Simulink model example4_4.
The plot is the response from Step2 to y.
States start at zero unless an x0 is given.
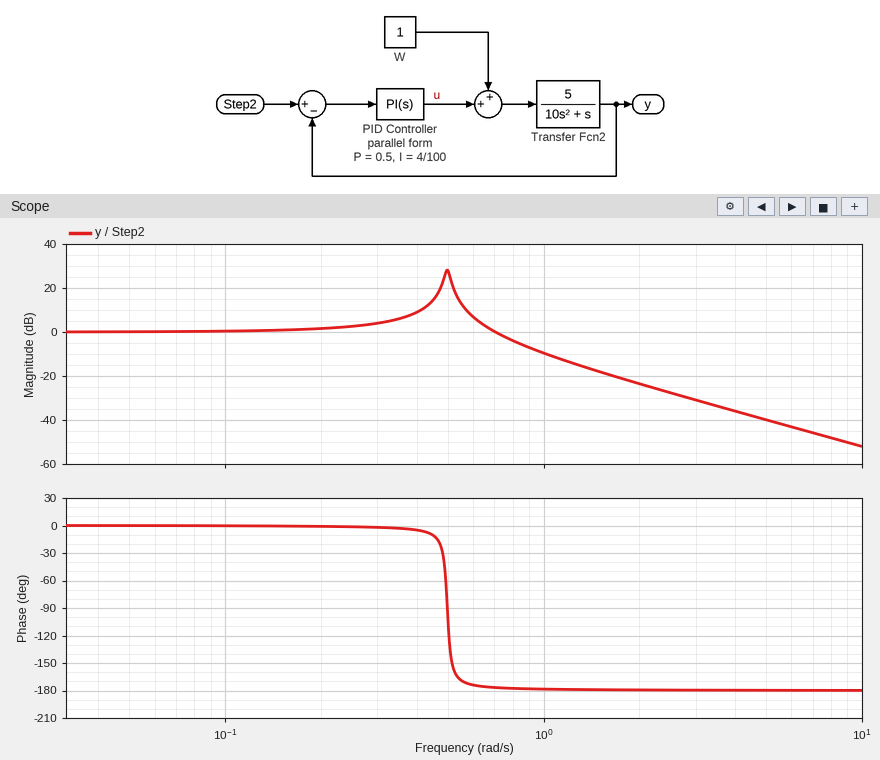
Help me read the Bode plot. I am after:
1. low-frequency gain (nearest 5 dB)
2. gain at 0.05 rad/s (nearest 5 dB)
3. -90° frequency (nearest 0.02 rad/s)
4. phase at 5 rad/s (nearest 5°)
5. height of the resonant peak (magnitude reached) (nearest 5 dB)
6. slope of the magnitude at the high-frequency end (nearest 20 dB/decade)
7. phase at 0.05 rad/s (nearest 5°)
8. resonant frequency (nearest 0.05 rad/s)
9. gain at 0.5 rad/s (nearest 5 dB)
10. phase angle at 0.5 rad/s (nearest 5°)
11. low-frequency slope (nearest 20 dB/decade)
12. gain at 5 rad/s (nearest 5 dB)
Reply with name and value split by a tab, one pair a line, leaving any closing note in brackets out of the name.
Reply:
low-frequency gain	0 dB
gain at 0.05 rad/s	0 dB
-90° frequency	0.50 rad/s
phase at 5 rad/s	-180°
height of the resonant peak (magnitude reached)	30 dB
slope of the magnitude at the high-frequency end	-40 dB/decade
phase at 0.05 rad/s	0°
resonant frequency	0.50 rad/s
gain at 0.5 rad/s	30 dB
phase angle at 0.5 rad/s	-100°
low-frequency slope	0 dB/decade
gain at 5 rad/s	-40 dB
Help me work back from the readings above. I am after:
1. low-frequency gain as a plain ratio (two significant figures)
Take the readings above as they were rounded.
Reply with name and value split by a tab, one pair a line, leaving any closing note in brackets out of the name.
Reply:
low-frequency gain as a plain ratio	1.0
